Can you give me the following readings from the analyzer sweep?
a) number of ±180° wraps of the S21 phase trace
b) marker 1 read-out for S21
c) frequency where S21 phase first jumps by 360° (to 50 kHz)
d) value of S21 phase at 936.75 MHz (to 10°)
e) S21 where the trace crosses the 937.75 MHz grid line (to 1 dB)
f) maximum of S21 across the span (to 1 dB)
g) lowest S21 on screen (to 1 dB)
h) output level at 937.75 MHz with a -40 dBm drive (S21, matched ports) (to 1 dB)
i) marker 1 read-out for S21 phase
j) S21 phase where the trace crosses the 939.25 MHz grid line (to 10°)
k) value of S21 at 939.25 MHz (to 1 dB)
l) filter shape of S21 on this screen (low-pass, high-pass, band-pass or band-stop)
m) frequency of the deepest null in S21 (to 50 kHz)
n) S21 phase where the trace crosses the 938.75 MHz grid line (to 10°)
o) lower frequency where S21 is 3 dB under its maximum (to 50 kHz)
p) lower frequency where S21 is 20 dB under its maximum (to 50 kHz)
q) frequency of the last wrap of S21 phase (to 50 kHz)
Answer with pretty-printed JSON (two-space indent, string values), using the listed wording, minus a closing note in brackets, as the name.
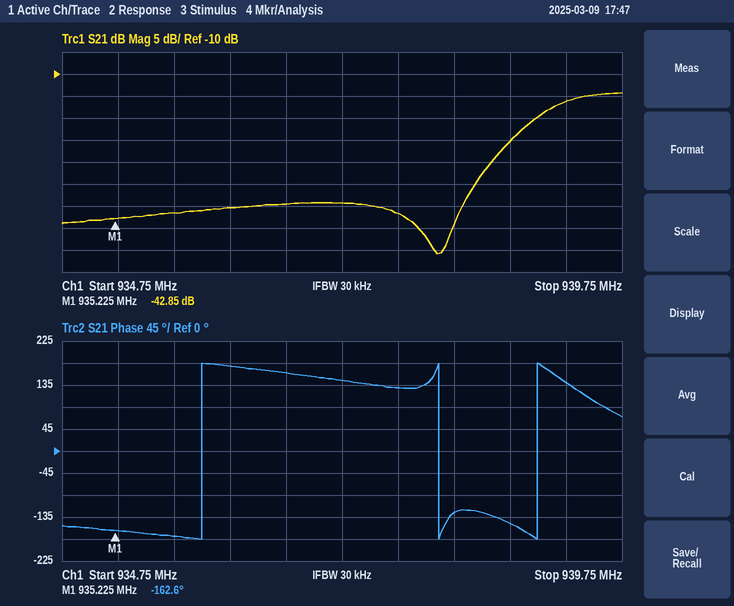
{
  "number of ±180° wraps of the S21 phase trace": "3",
  "marker 1 read-out for S21": "-42.85 dB",
  "frequency where S21 phase first jumps by 360°": "936.00 MHz",
  "value of S21 phase at 936.75 MHz": "160°",
  "S21 where the trace crosses the 937.75 MHz grid line": "-42 dB",
  "maximum of S21 across the span": "-14 dB",
  "lowest S21 on screen": "-51 dB",
  "output level at 937.75 MHz with a -40 dBm drive (S21, matched ports)": "-82 dBm",
  "marker 1 read-out for S21 phase": "-162.6°",
  "S21 phase where the trace crosses the 939.25 MHz grid line": "140°",
  "value of S21 at 939.25 MHz": "-16 dB",
  "filter shape of S21 on this screen": "high-pass",
  "frequency of the deepest null in S21": "938.10 MHz",
  "S21 phase where the trace crosses the 938.75 MHz grid line": "-150°",
  "lower frequency where S21 is 3 dB under its maximum": "939.15 MHz",
  "lower frequency where S21 is 20 dB under its maximum": "938.45 MHz",
  "frequency of the last wrap of S21 phase": "939.00 MHz"
}
